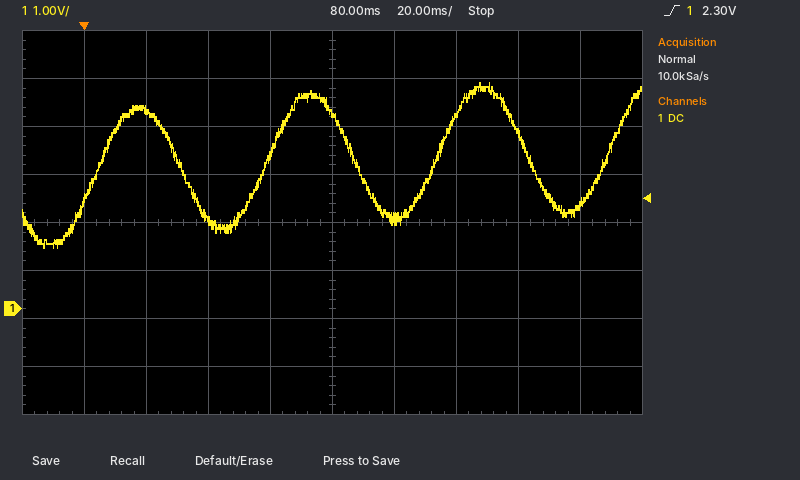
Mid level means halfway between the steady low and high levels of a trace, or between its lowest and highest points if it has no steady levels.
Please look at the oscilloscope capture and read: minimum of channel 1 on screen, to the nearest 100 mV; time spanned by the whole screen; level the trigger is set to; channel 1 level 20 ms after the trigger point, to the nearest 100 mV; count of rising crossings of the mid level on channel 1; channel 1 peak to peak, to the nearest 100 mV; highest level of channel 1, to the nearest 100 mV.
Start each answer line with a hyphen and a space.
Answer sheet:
- 1.3 V
- 200 ms
- 2.30 V
- 4.2 V
- 4
- 3.4 V
- 4.7 V
